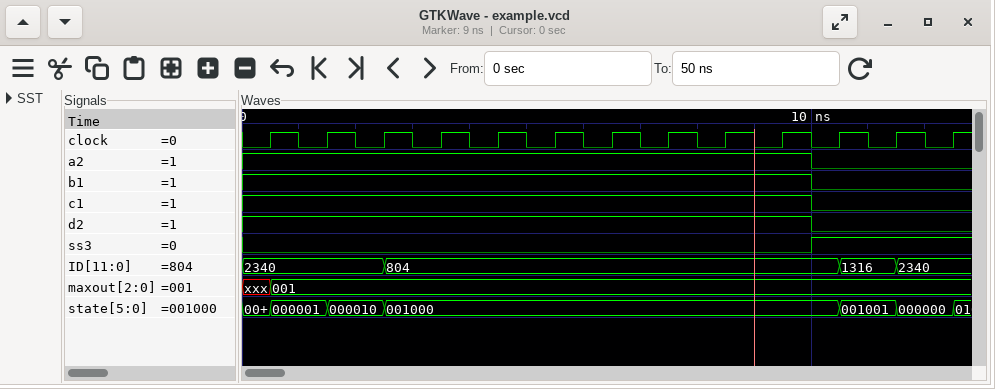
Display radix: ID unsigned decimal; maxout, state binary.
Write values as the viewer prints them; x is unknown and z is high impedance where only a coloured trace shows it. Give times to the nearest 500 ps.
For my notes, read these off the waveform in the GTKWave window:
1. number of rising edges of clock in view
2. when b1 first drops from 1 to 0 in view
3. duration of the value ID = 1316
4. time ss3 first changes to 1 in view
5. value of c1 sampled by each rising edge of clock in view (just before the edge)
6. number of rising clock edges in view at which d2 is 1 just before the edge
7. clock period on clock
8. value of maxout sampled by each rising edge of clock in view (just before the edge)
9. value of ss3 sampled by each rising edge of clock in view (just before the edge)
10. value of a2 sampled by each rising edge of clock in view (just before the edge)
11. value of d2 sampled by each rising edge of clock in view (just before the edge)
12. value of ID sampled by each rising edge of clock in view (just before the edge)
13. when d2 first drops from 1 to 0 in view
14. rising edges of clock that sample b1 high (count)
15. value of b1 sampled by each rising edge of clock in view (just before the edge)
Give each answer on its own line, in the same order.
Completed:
13
10000 ps
1000 ps
10000 ps
1 1 1 1 1 1 1 1 1 1 0 0 0
10
1000 ps
xxx, 001, 001, 001, 001, 001, 001, 001, 001, 001, 001, 001, 001
0 0 0 0 0 0 0 0 0 0 1 1 1
1 1 1 1 1 1 1 1 1 1 0 0 0
1 1 1 1 1 1 1 1 1 1 0 0 0
2340, 2340, 2340, 804, 804, 804, 804, 804, 804, 804, 804, 1316, 2340
10000 ps
10
1 1 1 1 1 1 1 1 1 1 0 0 0
